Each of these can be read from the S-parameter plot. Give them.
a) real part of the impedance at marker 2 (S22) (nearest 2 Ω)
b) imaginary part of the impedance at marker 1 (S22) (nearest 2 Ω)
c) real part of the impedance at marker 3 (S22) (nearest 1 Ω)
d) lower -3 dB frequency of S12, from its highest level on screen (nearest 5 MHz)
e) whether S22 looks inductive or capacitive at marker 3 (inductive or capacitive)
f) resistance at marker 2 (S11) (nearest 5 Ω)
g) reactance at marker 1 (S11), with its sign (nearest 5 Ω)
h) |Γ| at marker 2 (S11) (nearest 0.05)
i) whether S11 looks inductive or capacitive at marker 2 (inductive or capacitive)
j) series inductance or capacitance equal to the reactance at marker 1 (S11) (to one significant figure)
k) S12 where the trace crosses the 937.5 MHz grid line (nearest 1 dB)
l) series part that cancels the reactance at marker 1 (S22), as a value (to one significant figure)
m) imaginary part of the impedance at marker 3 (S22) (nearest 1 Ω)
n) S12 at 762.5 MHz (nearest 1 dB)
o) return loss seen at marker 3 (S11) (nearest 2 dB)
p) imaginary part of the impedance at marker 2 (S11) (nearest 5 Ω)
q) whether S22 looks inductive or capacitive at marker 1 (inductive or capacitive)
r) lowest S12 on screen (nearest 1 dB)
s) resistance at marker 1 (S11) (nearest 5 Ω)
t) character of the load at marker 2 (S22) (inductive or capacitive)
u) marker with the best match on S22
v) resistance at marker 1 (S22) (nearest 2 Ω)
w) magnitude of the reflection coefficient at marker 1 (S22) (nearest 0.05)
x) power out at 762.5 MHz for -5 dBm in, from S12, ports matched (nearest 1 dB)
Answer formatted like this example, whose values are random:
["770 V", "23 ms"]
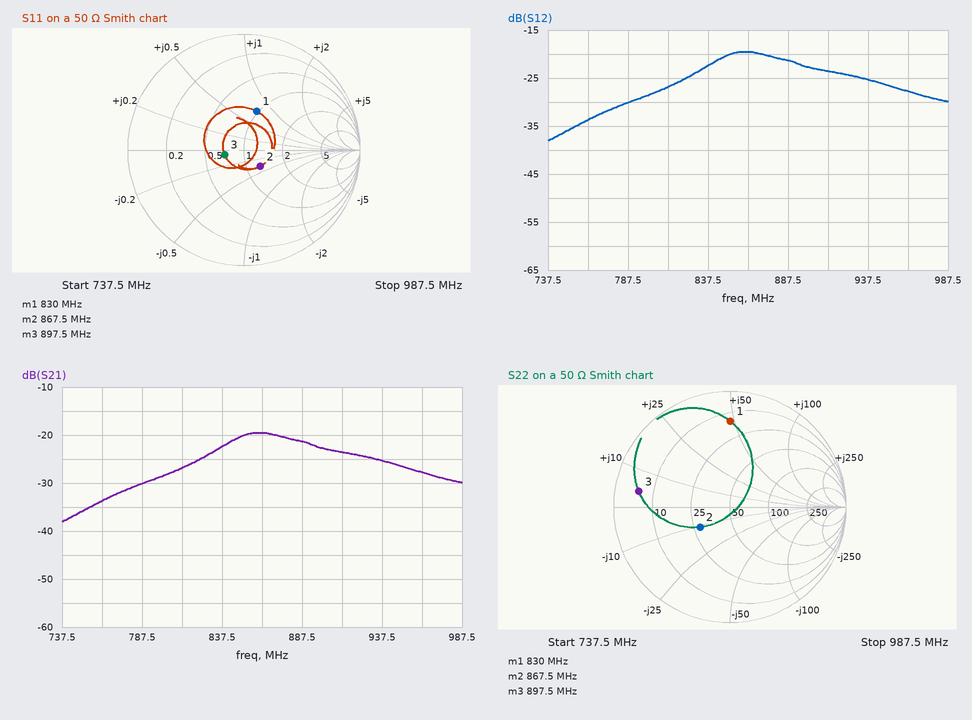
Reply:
["28 Ω", "+48 Ω", "6 Ω", "835 MHz", "inductive", "65 Ω", "+35 Ω", "0.20", "capacitive", "7 nH", "-25 dB", "4 pF", "+4 Ω", "-34 dB", "16 dB", "-20 Ω", "inductive", "-38 dB", "50 Ω", "capacitive", "marker 2", "14 Ω", "0.75", "-39 dBm"]
